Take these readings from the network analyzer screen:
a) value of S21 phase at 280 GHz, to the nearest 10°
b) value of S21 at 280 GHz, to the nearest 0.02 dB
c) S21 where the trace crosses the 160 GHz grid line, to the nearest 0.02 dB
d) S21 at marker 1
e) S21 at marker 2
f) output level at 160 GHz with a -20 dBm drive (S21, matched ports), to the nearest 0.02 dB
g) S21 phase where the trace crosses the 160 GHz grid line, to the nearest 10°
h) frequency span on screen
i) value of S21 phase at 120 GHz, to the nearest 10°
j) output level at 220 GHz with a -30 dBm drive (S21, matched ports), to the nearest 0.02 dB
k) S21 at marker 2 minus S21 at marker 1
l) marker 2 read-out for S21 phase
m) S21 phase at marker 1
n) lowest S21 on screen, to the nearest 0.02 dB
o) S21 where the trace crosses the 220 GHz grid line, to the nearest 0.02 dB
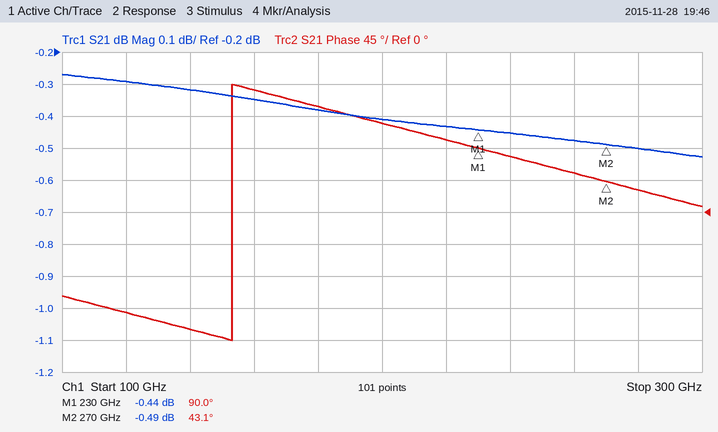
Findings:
30°
-0.50 dB
-0.34 dB
-0.44 dB
-0.49 dB
-20.34 dBm
170°
200 GHz
-140°
-30.44 dBm
-0.05 dB
43.1°
90.0°
-0.52 dB
-0.44 dB
